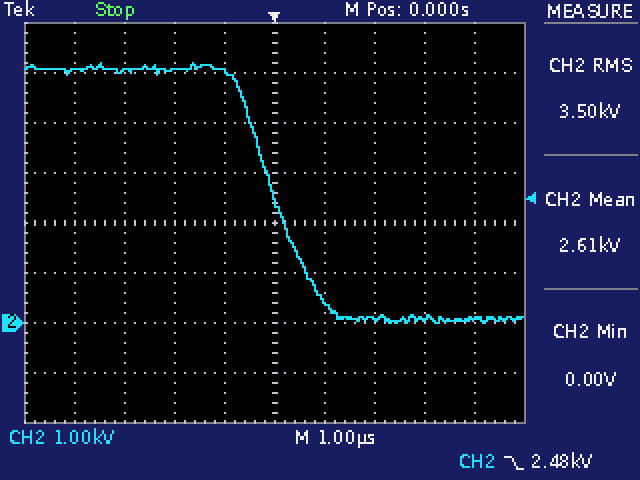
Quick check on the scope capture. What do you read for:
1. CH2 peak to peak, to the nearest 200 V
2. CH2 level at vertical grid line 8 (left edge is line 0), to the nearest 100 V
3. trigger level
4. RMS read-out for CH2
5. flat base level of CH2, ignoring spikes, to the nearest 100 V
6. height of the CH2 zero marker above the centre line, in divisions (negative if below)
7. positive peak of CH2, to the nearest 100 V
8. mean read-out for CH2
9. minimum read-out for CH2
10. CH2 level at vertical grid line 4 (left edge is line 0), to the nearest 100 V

5.2 kV
100 V
2.48 kV
3.50 kV
100 V
-2.0 div
5.2 kV
2.61 kV
0.00 V
5.0 kV
